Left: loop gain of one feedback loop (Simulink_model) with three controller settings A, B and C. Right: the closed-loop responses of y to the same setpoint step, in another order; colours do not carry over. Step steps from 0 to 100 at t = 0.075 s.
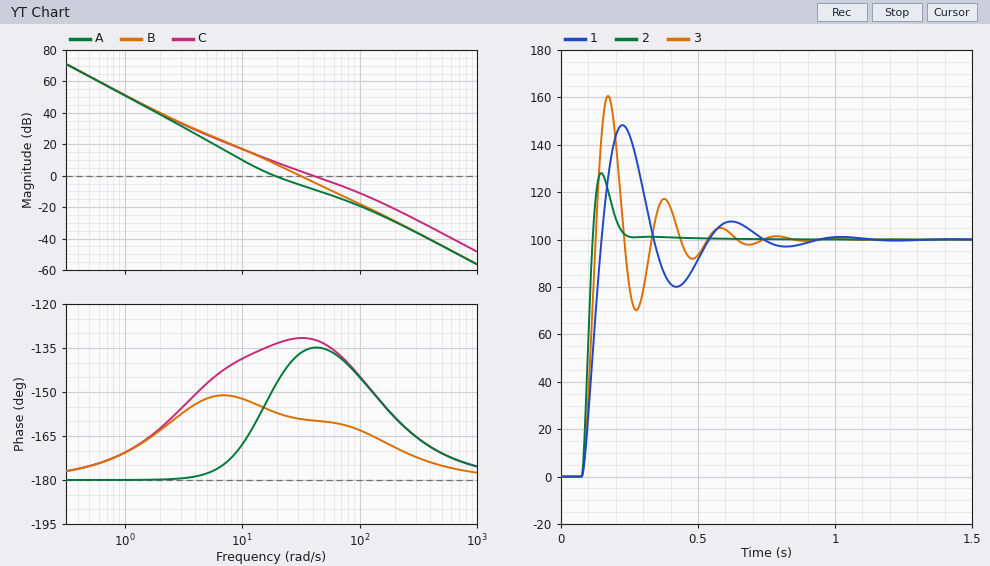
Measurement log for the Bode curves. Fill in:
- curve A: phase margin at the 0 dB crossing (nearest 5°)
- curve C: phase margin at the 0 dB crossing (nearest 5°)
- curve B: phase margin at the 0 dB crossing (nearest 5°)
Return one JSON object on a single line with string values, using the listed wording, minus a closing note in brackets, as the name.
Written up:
{"curve A: phase margin at the 0 dB crossing": "30°", "curve C: phase margin at the 0 dB crossing": "50°", "curve B: phase margin at the 0 dB crossing": "20°"}
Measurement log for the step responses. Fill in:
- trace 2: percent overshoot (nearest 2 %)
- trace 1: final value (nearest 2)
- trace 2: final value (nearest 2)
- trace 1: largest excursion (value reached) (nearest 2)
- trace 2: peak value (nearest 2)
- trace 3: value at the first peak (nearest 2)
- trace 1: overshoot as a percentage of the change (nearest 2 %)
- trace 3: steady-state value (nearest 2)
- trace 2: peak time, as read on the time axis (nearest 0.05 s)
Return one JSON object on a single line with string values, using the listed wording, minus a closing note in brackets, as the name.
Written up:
{"trace 2: percent overshoot": "28 %", "trace 1: final value": "100", "trace 2: final value": "100", "trace 1: largest excursion (value reached)": "148", "trace 2: peak value": "128", "trace 3: value at the first peak": "160", "trace 1: overshoot as a percentage of the change": "48 %", "trace 3: steady-state value": "100", "trace 2: peak time, as read on the time axis": "0.15 s"}
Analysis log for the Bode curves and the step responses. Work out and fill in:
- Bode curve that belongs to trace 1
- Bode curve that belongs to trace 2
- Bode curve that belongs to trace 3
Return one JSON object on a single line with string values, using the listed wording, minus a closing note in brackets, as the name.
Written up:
{"Bode curve that belongs to trace 1": "A", "Bode curve that belongs to trace 2": "C", "Bode curve that belongs to trace 3": "B"}
